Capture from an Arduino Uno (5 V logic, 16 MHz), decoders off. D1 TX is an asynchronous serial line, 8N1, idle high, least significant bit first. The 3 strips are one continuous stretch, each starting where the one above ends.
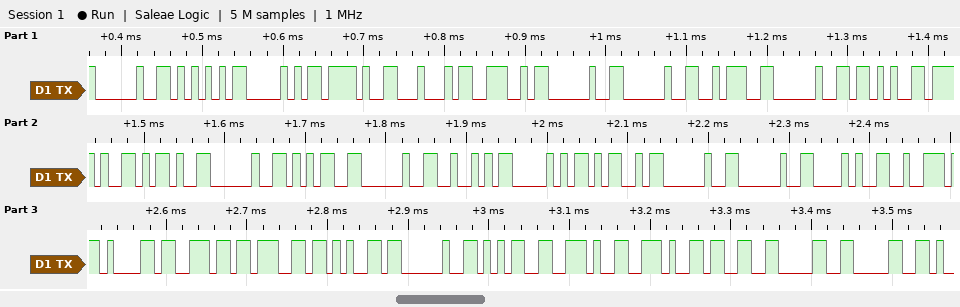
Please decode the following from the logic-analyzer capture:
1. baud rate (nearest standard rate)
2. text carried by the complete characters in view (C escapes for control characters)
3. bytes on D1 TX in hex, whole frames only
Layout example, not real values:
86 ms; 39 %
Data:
115200 baud; " UP/DN  : +/- 5 RPM  (range 5..300"; 0x20 0x55 0x50 0x2F 0x44 0x4E 0x20 0x20 0x3A 0x20 0x2B 0x2F 0x2D 0x20 0x35 0x20 0x52 0x50 0x4D 0x20 0x20 0x28 0x72 0x61 0x6E 0x67 0x65 0x20 0x35 0x2E 0x2E 0x33 0x30 0x30
